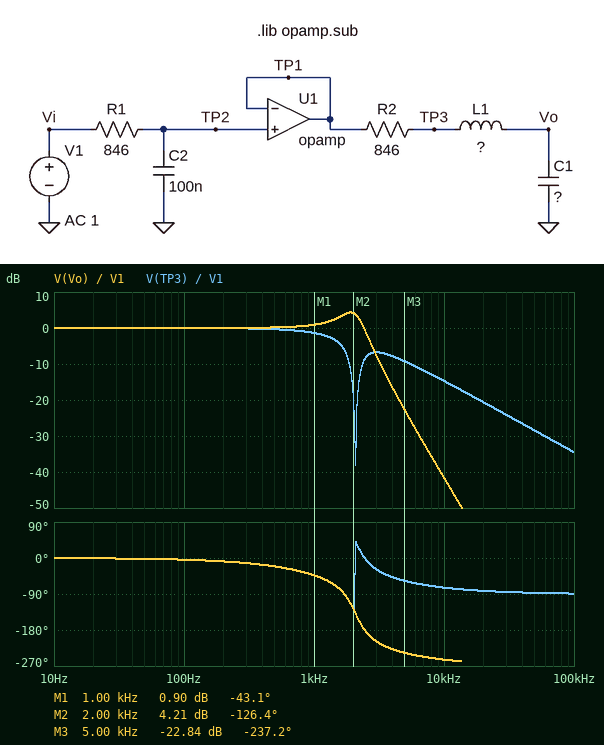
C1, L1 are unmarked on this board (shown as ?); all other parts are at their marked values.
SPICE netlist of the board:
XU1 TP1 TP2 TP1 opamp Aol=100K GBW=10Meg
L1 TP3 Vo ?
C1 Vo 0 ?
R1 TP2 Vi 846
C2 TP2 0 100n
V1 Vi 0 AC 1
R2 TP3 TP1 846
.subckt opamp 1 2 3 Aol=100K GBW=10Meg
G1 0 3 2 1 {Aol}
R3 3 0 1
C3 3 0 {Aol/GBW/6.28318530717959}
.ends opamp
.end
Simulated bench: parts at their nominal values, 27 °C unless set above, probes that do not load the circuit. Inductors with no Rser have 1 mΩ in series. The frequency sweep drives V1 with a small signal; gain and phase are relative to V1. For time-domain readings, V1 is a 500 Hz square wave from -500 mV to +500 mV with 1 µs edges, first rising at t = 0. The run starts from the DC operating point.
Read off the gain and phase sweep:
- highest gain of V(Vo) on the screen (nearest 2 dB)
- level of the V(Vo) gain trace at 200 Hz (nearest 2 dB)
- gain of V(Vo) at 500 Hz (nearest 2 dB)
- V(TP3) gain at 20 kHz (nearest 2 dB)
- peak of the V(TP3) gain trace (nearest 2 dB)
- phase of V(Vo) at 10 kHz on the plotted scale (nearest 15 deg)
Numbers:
4 dB
0 dB
0 dB
-20 dB
0 dB
-255 deg
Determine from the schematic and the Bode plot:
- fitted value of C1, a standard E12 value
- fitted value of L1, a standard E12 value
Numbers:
39 nF
150 mH
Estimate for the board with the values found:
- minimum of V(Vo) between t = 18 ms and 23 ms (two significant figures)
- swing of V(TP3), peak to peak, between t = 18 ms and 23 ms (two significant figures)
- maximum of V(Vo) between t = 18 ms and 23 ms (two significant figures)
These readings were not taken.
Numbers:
-770 mV
1.2 V
770 mV
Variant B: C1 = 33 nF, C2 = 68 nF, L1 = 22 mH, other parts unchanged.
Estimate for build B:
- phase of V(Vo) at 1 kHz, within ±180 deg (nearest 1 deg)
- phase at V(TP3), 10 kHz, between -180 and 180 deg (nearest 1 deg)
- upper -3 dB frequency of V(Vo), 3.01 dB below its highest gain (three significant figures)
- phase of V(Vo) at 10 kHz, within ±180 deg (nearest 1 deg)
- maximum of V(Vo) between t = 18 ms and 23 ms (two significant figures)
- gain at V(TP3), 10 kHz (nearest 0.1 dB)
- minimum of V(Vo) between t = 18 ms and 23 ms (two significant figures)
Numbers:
-30 deg
-31 deg
3.37 kHz
149 deg
500 mV
-14.2 dB
-500 mV
